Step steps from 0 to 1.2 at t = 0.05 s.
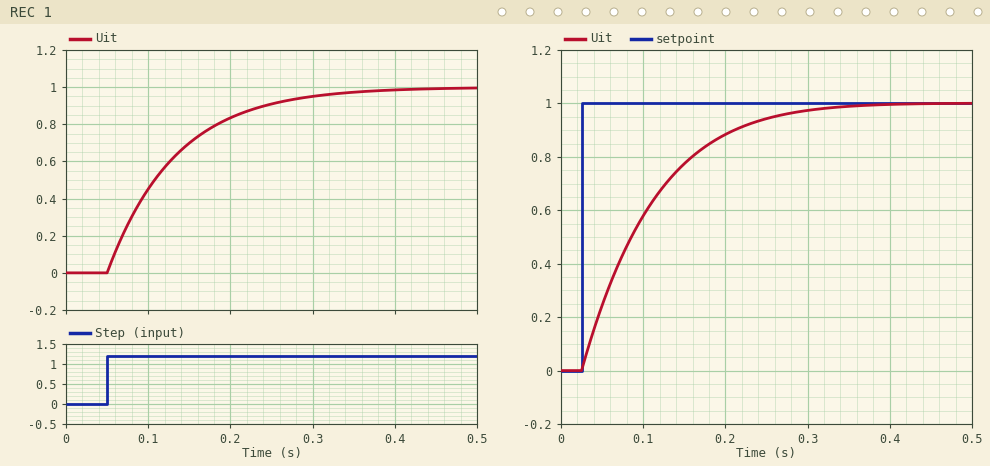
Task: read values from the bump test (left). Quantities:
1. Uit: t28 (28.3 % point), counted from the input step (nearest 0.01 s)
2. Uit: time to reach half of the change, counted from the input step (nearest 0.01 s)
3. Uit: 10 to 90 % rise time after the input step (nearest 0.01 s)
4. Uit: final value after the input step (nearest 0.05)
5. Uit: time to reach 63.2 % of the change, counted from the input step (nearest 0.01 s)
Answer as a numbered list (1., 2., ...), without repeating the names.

1. 0.03 s
2. 0.06 s
3. 0.18 s
4. 1.00
5. 0.08 s
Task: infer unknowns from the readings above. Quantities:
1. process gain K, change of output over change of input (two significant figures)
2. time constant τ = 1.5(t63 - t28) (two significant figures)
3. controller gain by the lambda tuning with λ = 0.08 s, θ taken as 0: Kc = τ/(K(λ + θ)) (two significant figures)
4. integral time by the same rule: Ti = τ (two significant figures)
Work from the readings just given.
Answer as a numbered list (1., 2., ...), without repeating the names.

1. 0.83
2. 0.075 s
3. 1.1
4. 0.075 s
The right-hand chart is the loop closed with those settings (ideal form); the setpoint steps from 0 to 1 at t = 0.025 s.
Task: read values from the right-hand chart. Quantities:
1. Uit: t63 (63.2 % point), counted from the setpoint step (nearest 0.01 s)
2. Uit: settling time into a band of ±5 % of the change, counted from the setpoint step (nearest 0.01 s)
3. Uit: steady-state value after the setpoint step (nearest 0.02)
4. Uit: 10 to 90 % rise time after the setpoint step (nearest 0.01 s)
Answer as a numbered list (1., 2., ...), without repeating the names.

1. 0.09 s
2. 0.23 s
3. 1.00
4. 0.18 s
